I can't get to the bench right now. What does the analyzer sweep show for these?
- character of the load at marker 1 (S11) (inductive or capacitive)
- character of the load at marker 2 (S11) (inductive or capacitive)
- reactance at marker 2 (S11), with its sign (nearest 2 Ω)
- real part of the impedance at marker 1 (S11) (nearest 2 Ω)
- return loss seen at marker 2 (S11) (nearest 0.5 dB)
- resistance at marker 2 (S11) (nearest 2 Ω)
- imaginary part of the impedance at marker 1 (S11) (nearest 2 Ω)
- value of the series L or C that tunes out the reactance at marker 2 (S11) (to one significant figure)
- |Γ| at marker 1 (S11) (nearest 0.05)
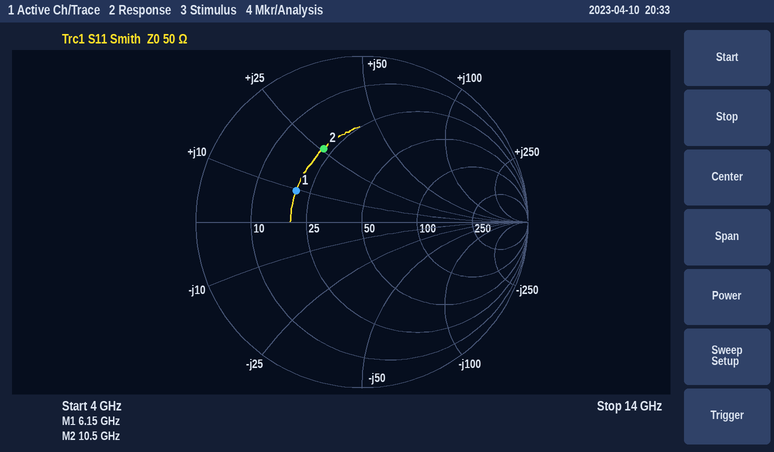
inductive
inductive
+26 Ω
20 Ω
6.0 dB
22 Ω
+10 Ω
600 fF
0.45
